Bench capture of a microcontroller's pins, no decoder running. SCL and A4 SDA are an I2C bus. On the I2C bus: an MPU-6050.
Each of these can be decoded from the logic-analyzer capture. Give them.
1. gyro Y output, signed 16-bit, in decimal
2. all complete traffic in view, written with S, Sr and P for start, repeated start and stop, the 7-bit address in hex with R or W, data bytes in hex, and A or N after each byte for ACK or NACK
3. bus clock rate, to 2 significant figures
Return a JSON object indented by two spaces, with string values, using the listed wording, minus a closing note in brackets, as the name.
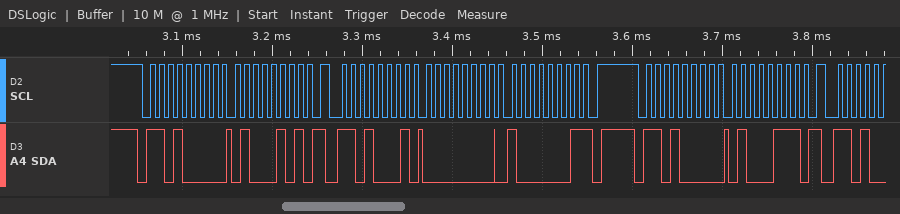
{
  "gyro Y output, signed 16-bit, in decimal": "129",
  "all complete traffic in view, written with S, Sr and P for start, repeated start and stop, the 7-bit address in hex with R or W, data bytes in hex, and A or N after each byte for ACK or NACK": "S 68W A 45 A Sr 68R A 00 A 81 N P S 68W A 47 A",
  "bus clock rate, to 2 significant figures": "100 kHz"
}
